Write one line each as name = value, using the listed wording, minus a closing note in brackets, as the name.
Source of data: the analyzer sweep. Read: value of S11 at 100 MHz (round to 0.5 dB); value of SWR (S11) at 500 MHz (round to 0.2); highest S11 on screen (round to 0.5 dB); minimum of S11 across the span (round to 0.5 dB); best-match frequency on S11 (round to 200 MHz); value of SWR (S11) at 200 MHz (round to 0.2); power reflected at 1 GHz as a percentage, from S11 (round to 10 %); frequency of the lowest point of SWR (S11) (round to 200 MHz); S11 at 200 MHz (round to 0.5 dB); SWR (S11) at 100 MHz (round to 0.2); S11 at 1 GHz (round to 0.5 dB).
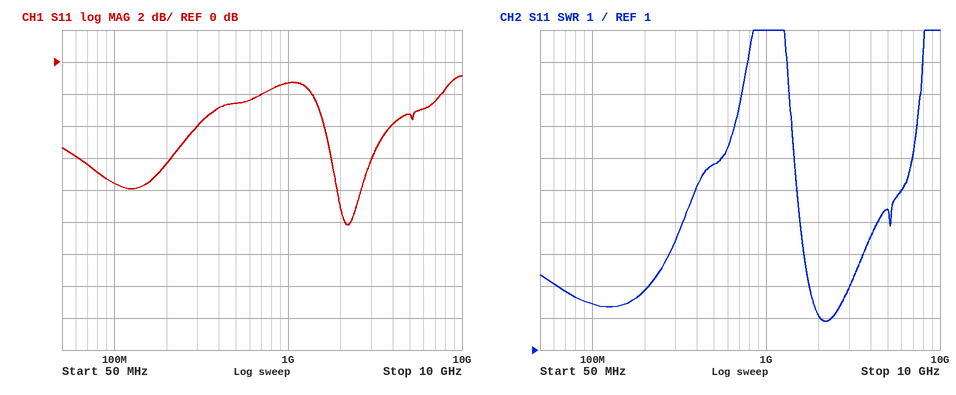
value of S11 at 100 MHz = -7.5 dB
value of SWR (S11) at 500 MHz = 6.8
highest S11 on screen = -1.0 dB
minimum of S11 across the span = -10.0 dB
best-match frequency on S11 = 2.2 GHz
value of SWR (S11) at 200 MHz = 2.8
power reflected at 1 GHz as a percentage, from S11 = 70 %
frequency of the lowest point of SWR (S11) = 2.2 GHz
S11 at 200 MHz = -6.5 dB
SWR (S11) at 100 MHz = 2.4
S11 at 1 GHz = -1.5 dB
